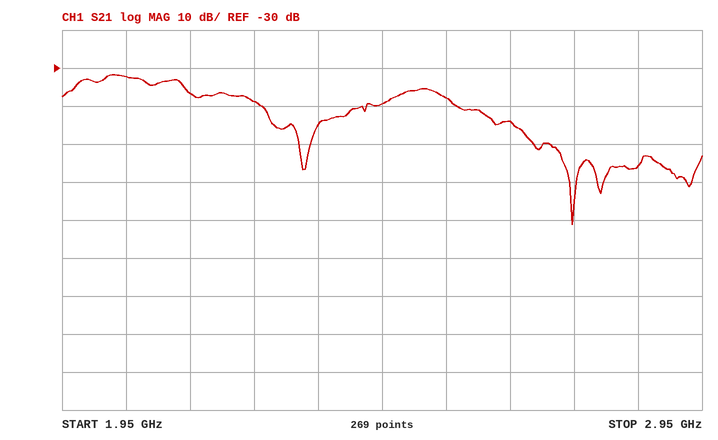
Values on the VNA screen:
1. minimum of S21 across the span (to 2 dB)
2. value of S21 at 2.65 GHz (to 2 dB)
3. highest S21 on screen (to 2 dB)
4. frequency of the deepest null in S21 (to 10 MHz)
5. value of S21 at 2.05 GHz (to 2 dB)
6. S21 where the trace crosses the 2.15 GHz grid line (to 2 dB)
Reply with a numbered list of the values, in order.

1. -72 dB
2. -44 dB
3. -32 dB
4. 2.75 GHz
5. -32 dB
6. -36 dB
